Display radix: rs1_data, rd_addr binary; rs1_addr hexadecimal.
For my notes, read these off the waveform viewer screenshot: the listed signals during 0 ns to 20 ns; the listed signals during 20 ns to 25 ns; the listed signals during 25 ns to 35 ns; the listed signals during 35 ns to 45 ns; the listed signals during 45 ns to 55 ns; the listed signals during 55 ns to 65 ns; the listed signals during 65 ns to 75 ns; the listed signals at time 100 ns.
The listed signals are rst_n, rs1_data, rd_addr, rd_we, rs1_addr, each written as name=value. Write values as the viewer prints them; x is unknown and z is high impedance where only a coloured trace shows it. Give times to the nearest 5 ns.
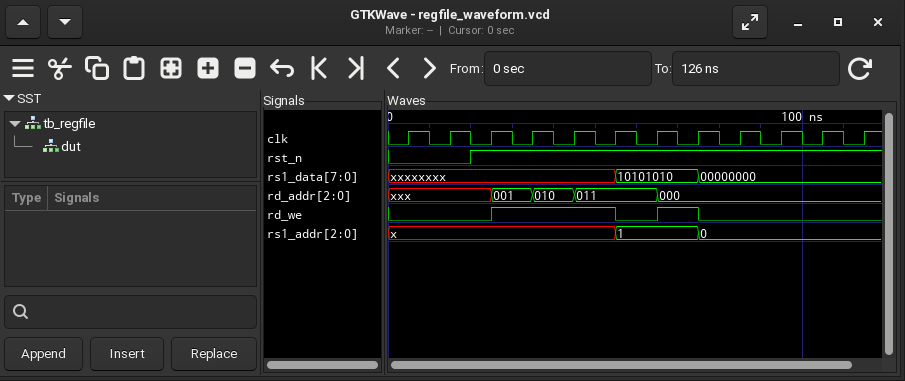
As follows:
rst_n=0, rs1_data=xxxxxxxx, rd_addr=xxx, rd_we=0, rs1_addr=x
rst_n=1, rs1_data=xxxxxxxx, rd_addr=xxx, rd_we=0, rs1_addr=x
rst_n=1, rs1_data=xxxxxxxx, rd_addr=001, rd_we=1, rs1_addr=x
rst_n=1, rs1_data=xxxxxxxx, rd_addr=010, rd_we=1, rs1_addr=x
rst_n=1, rs1_data=xxxxxxxx, rd_addr=011, rd_we=1, rs1_addr=x
rst_n=1, rs1_data=10101010, rd_addr=011, rd_we=0, rs1_addr=1
rst_n=1, rs1_data=10101010, rd_addr=000, rd_we=1, rs1_addr=1
rst_n=1, rs1_data=00000000, rd_addr=000, rd_we=0, rs1_addr=0
